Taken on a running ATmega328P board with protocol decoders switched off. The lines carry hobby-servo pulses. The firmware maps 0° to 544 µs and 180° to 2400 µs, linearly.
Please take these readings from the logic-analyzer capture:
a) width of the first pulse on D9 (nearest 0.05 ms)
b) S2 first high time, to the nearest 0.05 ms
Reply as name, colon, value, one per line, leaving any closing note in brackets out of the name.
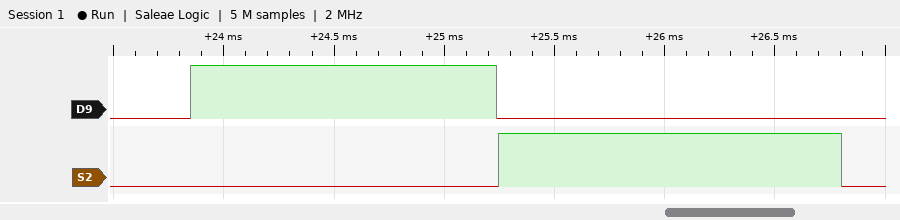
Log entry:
width of the first pulse on D9: 1.40 ms
S2 first high time, to the nearest 0.05 ms: 1.55 ms
